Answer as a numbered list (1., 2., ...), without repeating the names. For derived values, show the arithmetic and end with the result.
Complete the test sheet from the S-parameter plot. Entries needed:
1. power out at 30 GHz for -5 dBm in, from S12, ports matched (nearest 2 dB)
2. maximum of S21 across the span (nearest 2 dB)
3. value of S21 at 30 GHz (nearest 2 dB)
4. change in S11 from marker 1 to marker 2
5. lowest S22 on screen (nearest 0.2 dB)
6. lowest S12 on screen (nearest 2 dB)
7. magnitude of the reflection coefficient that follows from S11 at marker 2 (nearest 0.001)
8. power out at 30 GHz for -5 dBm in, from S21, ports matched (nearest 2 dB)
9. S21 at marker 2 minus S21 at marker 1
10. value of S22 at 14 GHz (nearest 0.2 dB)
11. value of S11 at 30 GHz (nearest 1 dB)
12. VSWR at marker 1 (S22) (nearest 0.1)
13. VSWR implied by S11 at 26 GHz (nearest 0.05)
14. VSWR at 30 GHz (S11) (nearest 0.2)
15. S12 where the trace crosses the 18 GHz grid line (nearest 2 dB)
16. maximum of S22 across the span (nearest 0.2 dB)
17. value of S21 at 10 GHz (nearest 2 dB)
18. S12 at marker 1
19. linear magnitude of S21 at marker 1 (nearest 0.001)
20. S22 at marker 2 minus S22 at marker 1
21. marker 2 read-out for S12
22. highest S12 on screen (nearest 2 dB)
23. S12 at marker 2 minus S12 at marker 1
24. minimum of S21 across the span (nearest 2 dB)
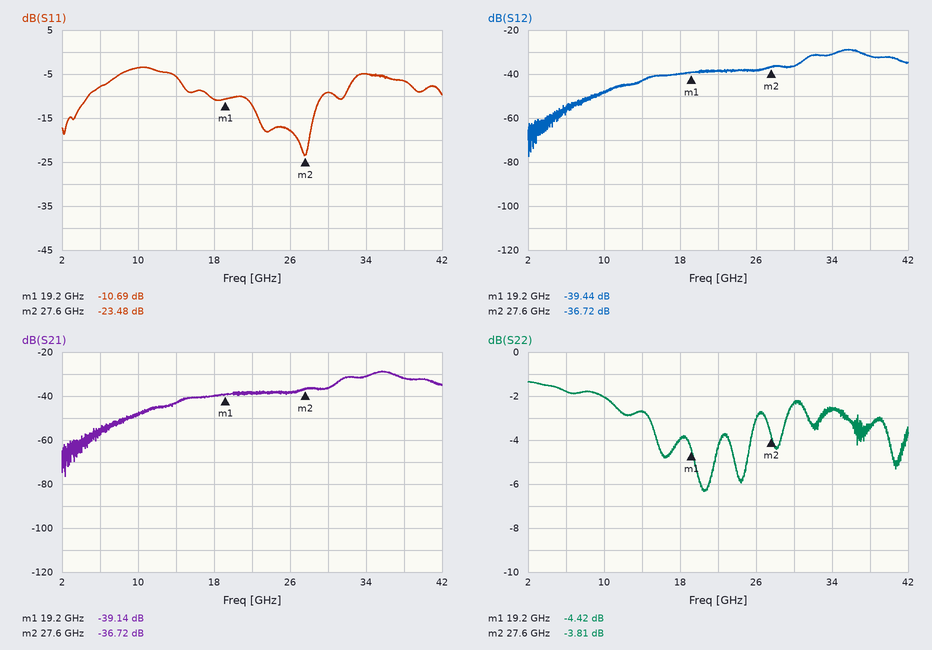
1. -5 dBm + (-36 dB) = -42 dBm
2. -28 dB
3. -36 dB
4. -23.48 − (-10.69) = -12.79 dB
5. -6.4 dB
6. -78 dB
7. 10^(-23.48/20) ≈ 0.067
8. -5 dBm + (-36 dB) = -42 dBm
9. -36.72 − (-39.14) = 2.42 dB
10. -2.6 dB
11. -9 dB
12. (1 + 0.6012)/(1 − 0.6012) ≈ 4.0
13. |Γ| = 10^(-18/20) = 0.1259; VSWR = (1 + 0.1259)/(1 − 0.1259) ≈ 1.29, so 1.30 to the nearest 0.05
14. |Γ| = 10^(-9/20) = 0.3548; VSWR = (1 + 0.3548)/(1 − 0.3548) ≈ 2.10, so 2.0 to the nearest 0.2
15. -40 dB
16. -1.4 dB
17. -48 dB
18. -39.44 dB
19. 10^(-39.14/20) ≈ 0.011
20. -3.81 − (-4.42) = 0.61 dB
21. -36.72 dB
22. -28 dB
23. -36.72 − (-39.44) = 2.72 dB
24. -76 dB
